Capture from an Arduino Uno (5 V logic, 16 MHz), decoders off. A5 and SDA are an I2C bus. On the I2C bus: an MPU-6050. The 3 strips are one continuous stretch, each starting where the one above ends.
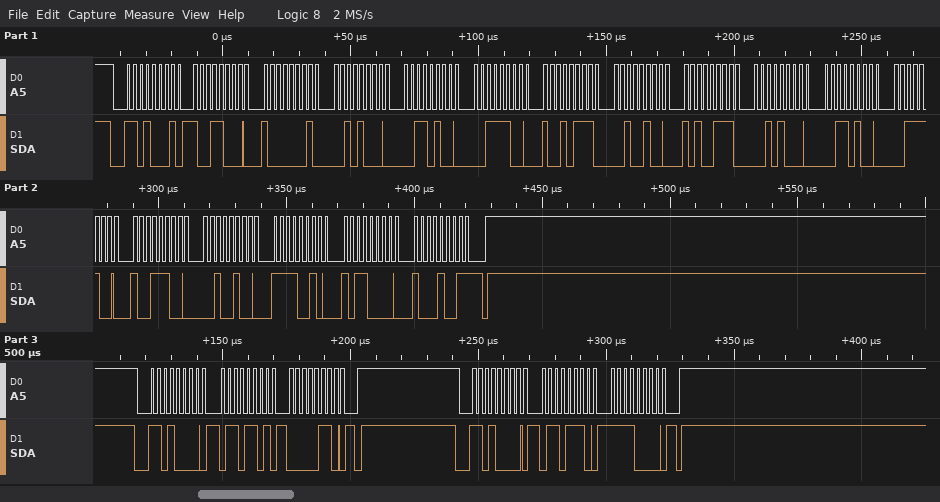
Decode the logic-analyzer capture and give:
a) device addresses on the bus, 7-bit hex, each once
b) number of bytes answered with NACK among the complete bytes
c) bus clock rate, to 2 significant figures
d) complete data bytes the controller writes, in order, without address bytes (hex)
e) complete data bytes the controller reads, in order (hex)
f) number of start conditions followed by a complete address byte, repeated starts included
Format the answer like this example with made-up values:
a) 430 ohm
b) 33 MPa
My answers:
a) 0x68
b) 1
c) 400 kHz
d) 6D 06 6E F0
e) 98 81 28 34 3C 97 24 A7 28 34 3C 9C 24 F2 B0 89
f) 3
